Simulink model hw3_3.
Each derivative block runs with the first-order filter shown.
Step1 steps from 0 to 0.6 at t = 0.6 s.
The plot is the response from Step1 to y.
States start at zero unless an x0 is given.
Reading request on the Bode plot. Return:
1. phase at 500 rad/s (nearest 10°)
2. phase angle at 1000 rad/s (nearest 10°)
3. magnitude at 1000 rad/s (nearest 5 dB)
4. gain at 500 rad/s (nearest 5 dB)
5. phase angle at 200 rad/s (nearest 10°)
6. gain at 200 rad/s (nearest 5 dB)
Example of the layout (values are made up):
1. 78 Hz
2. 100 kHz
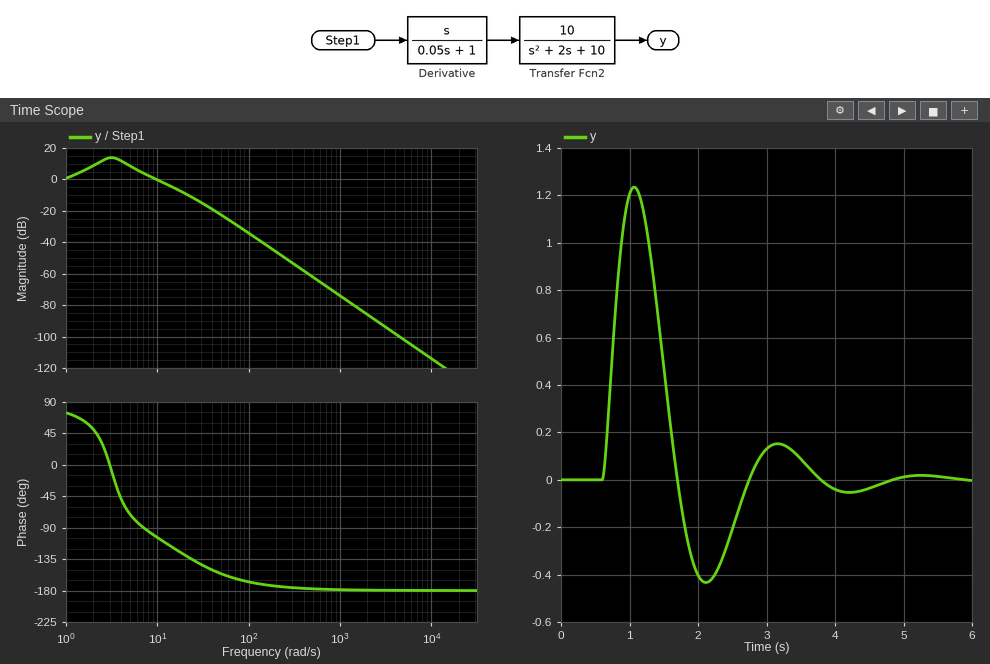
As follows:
1. -180°
2. -180°
3. -75 dB
4. -60 dB
5. -170°
6. -45 dB
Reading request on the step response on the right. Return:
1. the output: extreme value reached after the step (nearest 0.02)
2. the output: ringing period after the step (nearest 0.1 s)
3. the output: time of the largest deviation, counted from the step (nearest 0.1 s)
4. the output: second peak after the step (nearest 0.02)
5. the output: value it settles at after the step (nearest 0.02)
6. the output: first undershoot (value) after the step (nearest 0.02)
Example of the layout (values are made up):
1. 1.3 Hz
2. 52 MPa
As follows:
1. 1.24
2. 2.1 s
3. 0.5 s
4. 0.16
5. 0.00
6. -0.44
